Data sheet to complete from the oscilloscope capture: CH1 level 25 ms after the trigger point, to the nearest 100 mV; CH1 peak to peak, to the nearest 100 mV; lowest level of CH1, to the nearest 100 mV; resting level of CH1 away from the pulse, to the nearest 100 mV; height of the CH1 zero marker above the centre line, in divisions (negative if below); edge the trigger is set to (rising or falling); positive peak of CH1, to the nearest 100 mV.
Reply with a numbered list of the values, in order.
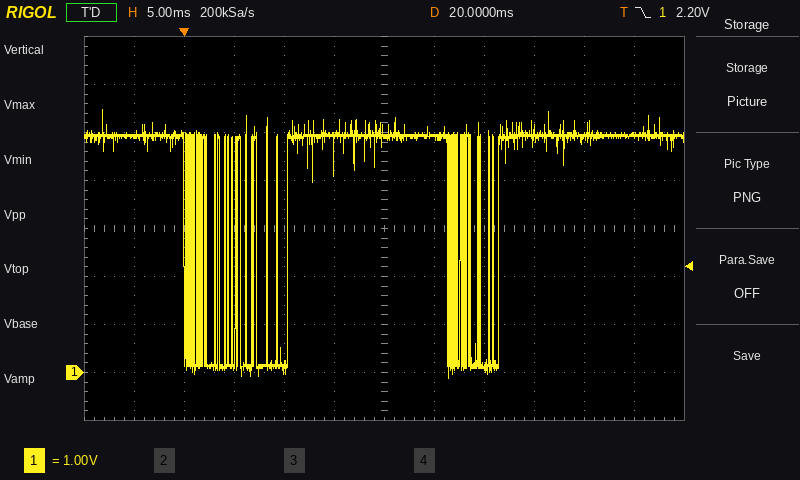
1. 4.9 V
2. 5.6 V
3. -100 mV
4. 4.9 V
5. -3.0 div
6. falling
7. 5.5 V
